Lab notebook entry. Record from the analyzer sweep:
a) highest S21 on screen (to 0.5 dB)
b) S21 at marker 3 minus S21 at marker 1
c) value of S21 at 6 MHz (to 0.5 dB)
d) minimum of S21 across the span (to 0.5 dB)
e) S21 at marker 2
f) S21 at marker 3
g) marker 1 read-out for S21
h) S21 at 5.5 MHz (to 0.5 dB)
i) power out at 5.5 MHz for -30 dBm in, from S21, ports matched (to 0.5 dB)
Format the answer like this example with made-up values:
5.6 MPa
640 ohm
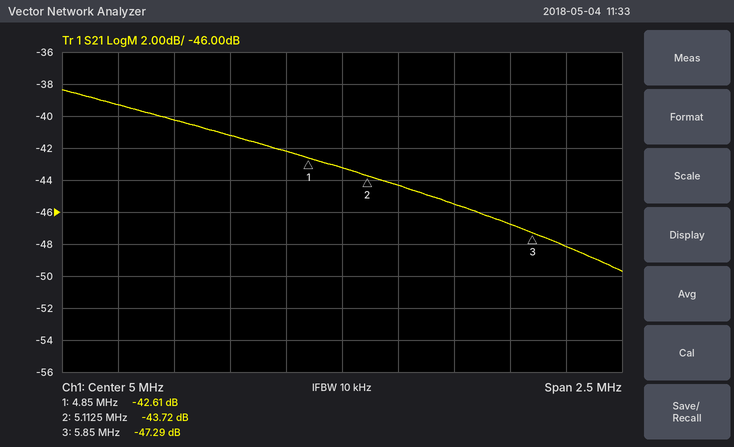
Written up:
-38.5 dB
-4.68 dB
-48.0 dB
-49.5 dB
-43.72 dB
-47.29 dB
-42.61 dB
-45.5 dB
-75.5 dBm
